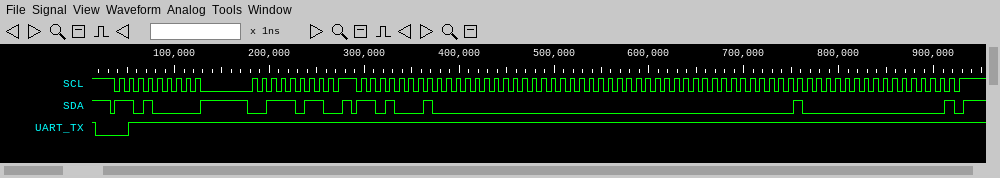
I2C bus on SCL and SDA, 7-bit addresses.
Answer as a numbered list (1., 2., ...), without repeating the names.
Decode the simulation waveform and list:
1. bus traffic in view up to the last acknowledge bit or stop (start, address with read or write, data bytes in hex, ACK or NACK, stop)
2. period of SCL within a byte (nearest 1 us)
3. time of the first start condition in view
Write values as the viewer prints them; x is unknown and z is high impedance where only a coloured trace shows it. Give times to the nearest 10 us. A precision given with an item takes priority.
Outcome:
1. start, address 68 write ACK, 3B ACK, stop, start, address 68 read ACK, 00 ACK, 00 ACK, 00 ACK, 00 ACK, 40 ACK, 00 NACK, stop
2. 10 us
3. 30 us
